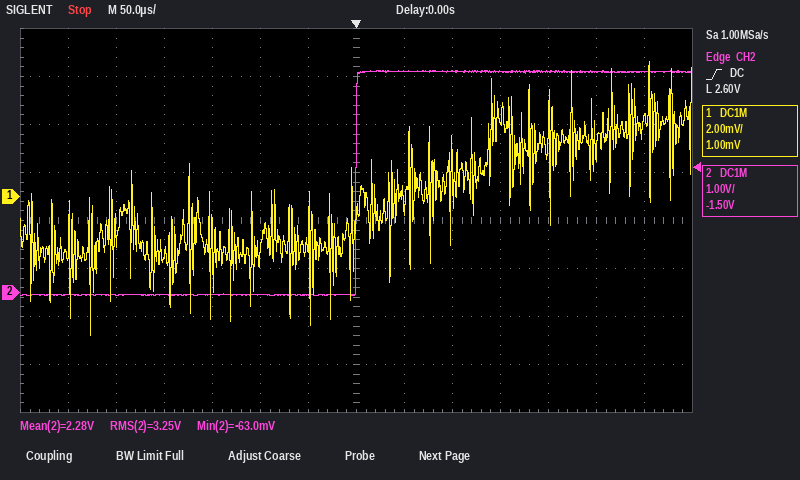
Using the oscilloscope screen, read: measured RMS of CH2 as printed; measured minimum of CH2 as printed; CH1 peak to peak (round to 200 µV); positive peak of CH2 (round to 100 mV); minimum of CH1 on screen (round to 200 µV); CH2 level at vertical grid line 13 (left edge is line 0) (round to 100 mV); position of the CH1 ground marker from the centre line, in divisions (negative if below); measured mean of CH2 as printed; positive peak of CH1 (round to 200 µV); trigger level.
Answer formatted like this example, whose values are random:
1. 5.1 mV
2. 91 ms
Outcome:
1. 3.25 V
2. -63.0 mV
3. 11.4 mV
4. 4.6 V
5. -5.8 mV
6. 4.6 V
7. +0.5 div
8. 2.28 V
9. 5.6 mV
10. 2.60 V
